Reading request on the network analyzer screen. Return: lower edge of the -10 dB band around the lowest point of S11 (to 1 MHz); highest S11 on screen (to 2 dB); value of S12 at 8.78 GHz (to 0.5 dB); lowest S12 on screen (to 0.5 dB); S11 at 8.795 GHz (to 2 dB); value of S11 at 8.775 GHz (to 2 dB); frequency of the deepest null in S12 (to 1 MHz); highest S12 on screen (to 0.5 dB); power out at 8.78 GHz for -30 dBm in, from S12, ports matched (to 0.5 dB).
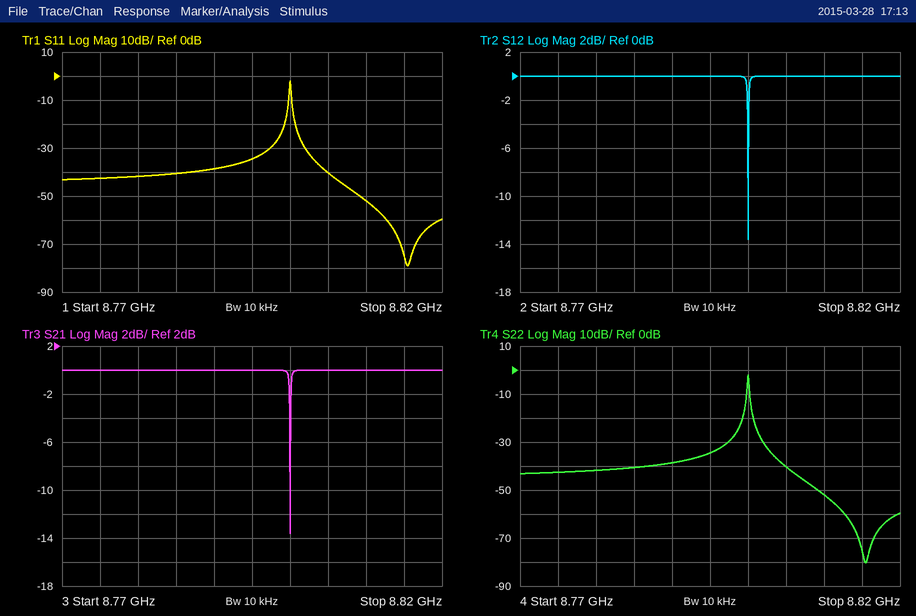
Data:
8.800 GHz
-2 dB
0.0 dB
-13.5 dB
-34 dB
-42 dB
8.800 GHz
0.0 dB
-30.0 dBm
